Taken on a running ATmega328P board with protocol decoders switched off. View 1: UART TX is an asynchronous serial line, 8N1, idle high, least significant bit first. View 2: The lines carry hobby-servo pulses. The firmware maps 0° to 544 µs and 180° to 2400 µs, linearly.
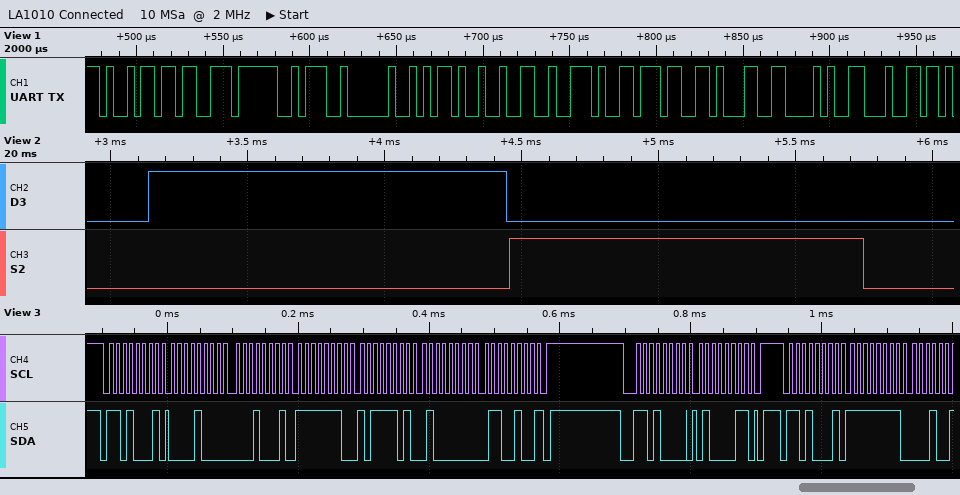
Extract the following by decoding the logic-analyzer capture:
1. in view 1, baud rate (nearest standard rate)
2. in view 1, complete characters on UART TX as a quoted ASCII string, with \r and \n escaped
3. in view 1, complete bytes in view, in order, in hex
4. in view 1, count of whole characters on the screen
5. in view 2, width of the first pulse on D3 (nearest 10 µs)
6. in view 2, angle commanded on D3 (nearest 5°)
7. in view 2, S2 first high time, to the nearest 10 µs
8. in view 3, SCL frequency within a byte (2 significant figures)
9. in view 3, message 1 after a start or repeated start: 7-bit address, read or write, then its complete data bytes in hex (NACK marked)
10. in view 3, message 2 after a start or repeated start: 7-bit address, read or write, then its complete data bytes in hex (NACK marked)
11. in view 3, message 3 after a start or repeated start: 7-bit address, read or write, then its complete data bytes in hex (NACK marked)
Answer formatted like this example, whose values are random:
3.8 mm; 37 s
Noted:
250000 baud; "is: -2.71(d"; 69 73 3A 20 2D 32 2E 37 31 28 64; 11; 1310 µs; 75°; 1290 µs; 100 kHz; 0x68 read: 08 11 FE BD 40 64 NACK; 0x68 write: 43; 0x68 read: FF
